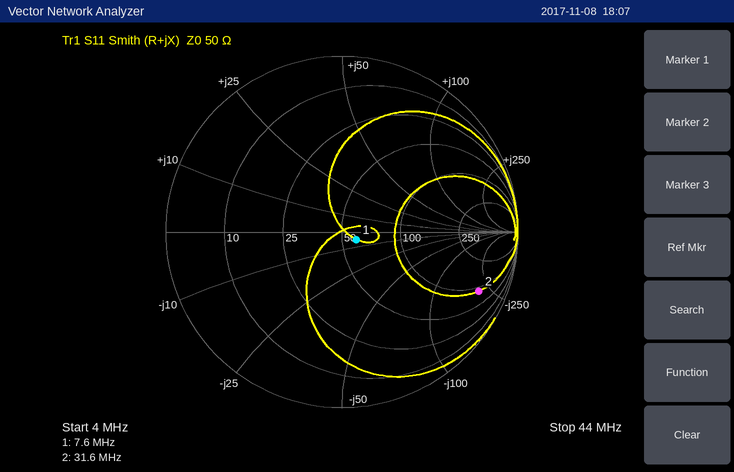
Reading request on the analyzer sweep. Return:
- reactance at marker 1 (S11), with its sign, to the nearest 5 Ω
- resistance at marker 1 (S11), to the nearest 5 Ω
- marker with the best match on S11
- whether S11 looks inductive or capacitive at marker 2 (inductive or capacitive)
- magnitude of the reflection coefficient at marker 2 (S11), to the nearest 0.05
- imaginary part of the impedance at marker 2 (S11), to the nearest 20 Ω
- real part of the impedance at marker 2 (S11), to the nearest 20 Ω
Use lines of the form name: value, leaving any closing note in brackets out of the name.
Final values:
reactance at marker 1 (S11), with its sign, to the nearest 5 Ω: -5 Ω
resistance at marker 1 (S11), to the nearest 5 Ω: 60 Ω
marker with the best match on S11: marker 1
whether S11 looks inductive or capacitive at marker 2: capacitive
magnitude of the reflection coefficient at marker 2 (S11), to the nearest 0.05: 0.85
imaginary part of the impedance at marker 2 (S11), to the nearest 20 Ω: -200 Ω
real part of the impedance at marker 2 (S11), to the nearest 20 Ω: 80 Ω
